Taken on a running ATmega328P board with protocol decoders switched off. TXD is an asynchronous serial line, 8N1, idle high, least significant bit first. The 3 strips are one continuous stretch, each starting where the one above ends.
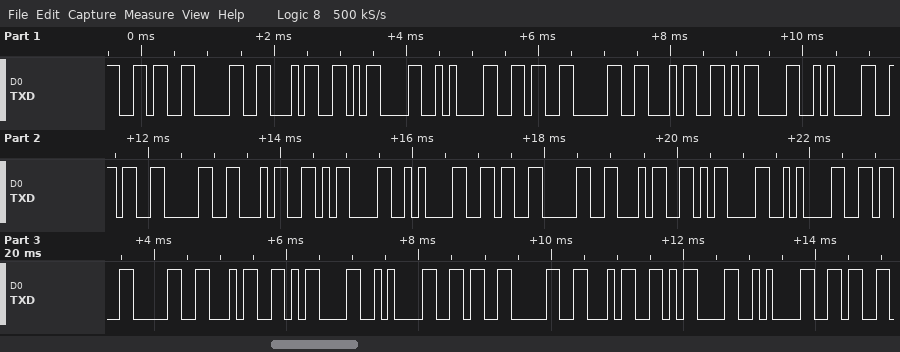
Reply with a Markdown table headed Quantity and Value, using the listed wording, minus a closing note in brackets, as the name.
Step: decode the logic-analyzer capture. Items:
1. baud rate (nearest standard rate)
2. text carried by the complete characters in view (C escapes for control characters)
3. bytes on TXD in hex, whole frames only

| Quantity | Value |
|---|---|
| baud rate | 9600 baud |
| text carried by the complete characters in view | "604\r\n604\r\n604\r\n604\r\n604\r\n604\r\n6" |
| bytes on TXD in hex, whole frames only | 36 30 34 0D 0A 36 30 34 0D 0A 36 30 34 0D 0A 36 30 34 0D 0A 36 30 34 0D 0A 36 30 34 0D 0A 36 |
